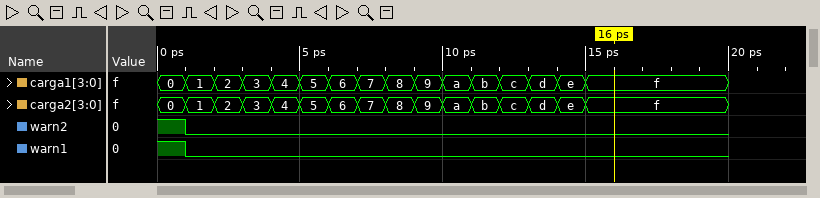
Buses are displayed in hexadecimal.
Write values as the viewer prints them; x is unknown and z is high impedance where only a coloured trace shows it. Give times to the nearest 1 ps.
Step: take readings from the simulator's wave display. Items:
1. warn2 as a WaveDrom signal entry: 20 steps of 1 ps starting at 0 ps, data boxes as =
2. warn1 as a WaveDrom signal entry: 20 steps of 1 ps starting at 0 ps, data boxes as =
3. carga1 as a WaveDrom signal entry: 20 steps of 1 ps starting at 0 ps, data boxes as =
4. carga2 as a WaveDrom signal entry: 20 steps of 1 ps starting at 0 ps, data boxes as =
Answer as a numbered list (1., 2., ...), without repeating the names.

1. {name: 'warn2', wave: '10..................'}
2. {name: 'warn1', wave: '10..................'}
3. {name: 'carga1', wave: '================....', data: '0 1 2 3 4 5 6 7 8 9 a b c d e f'}
4. {name: 'carga2', wave: '================....', data: '0 1 2 3 4 5 6 7 8 9 a b c d e f'}
